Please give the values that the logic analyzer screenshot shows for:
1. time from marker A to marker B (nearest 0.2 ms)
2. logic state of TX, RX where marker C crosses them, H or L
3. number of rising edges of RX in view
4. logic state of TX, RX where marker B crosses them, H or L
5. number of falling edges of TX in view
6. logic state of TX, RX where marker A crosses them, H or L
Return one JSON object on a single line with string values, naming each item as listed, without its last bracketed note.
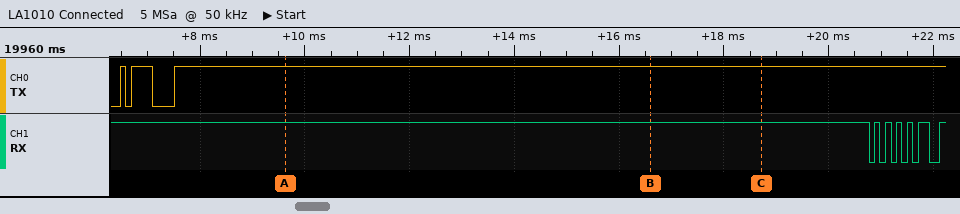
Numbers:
{"time from marker A to marker B": "7 ms", "logic state of TX, RX where marker C crosses them, H or L": "TX=H, RX=H", "number of rising edges of RX in view": "6", "logic state of TX, RX where marker B crosses them, H or L": "TX=H, RX=H", "number of falling edges of TX in view": "2", "logic state of TX, RX where marker A crosses them, H or L": "TX=H, RX=H"}
